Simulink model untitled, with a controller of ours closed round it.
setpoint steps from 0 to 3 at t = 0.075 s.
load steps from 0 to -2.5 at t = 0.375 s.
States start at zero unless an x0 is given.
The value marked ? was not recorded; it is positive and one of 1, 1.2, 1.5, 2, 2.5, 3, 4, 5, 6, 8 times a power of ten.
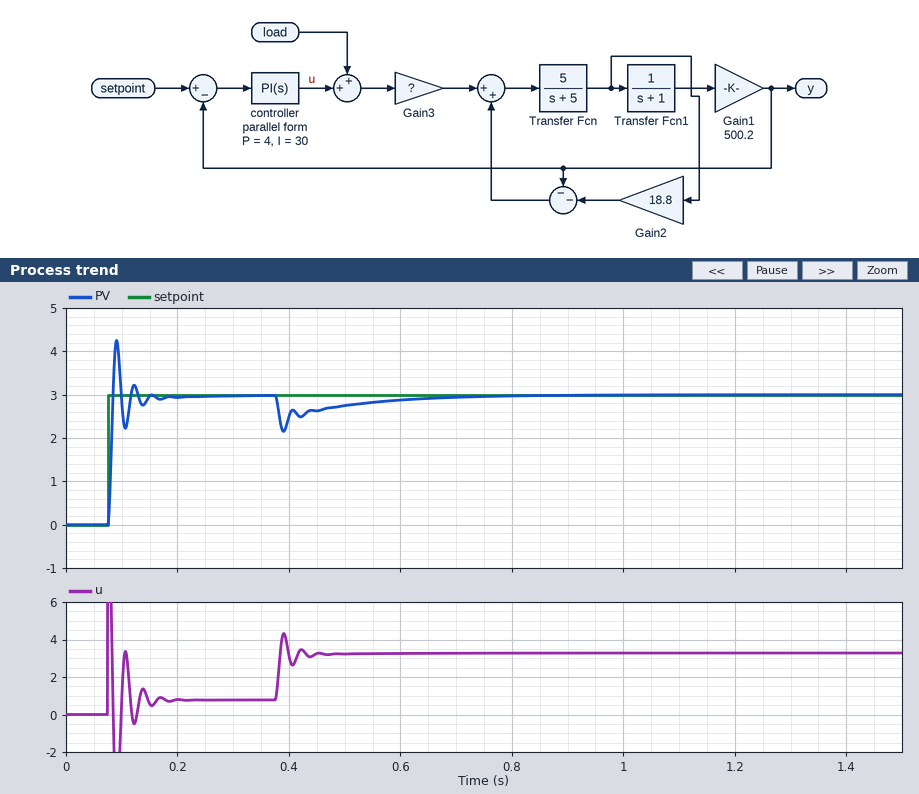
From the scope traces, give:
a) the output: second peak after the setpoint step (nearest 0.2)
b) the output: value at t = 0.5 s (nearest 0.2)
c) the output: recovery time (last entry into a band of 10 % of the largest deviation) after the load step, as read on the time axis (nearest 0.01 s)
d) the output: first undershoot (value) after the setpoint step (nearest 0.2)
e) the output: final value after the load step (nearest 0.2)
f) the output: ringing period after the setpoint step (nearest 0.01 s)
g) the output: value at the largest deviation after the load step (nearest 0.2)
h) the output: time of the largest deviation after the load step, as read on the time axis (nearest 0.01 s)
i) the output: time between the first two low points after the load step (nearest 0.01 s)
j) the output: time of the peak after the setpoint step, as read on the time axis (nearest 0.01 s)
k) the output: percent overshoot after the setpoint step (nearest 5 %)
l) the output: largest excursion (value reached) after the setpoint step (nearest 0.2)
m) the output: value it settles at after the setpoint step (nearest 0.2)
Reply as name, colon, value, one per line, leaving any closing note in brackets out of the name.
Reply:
the output: second peak after the setpoint step: 3.2
the output: value at t = 0.5 s: 2.8
the output: recovery time (last entry into a band of 10 % of the largest deviation) after the load step, as read on the time axis: 0.66 s
the output: first undershoot (value) after the setpoint step: 2.2
the output: final value after the load step: 3.0
the output: ringing period after the setpoint step: 0.03 s
the output: value at the largest deviation after the load step: 2.2
the output: time of the largest deviation after the load step, as read on the time axis: 0.39 s
the output: time between the first two low points after the load step: 0.03 s
the output: time of the peak after the setpoint step, as read on the time axis: 0.09 s
the output: percent overshoot after the setpoint step: 40 %
the output: largest excursion (value reached) after the setpoint step: 4.2
the output: value it settles at after the setpoint step: 3.0
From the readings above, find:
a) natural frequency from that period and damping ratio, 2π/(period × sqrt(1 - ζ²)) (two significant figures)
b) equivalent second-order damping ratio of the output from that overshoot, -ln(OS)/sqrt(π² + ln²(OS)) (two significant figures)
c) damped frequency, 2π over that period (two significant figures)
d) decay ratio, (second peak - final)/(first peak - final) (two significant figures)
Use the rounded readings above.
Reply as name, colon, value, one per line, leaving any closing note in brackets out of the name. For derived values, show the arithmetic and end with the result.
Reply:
natural frequency from that period and damping ratio, 2π/(period × sqrt(1 - ζ²)): 2π / (0.03 × sqrt(1 - 0.28²)) = 220 rad/s
equivalent second-order damping ratio of the output from that overshoot, -ln(OS)/sqrt(π² + ln²(OS)): ln(0.4) = -0.916; 0.916 / sqrt(9.870 + 0.840) = 0.28
damped frequency, 2π over that period: 2π / 0.03 = 210 rad/s
decay ratio, (second peak - final)/(first peak - final): (3.2 - 3) / (4.2 - 3) = 0.17
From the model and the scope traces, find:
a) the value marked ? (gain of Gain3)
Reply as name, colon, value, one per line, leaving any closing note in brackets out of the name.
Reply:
the value marked ?: 4
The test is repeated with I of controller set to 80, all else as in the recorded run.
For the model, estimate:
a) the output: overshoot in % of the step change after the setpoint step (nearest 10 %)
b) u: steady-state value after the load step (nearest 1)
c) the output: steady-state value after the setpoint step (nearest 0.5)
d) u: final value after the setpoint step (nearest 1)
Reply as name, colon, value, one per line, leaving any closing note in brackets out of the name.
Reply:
the output: overshoot in % of the step change after the setpoint step: 50 %
u: steady-state value after the load step: 3
the output: steady-state value after the setpoint step: 3.0
u: final value after the setpoint step: 1
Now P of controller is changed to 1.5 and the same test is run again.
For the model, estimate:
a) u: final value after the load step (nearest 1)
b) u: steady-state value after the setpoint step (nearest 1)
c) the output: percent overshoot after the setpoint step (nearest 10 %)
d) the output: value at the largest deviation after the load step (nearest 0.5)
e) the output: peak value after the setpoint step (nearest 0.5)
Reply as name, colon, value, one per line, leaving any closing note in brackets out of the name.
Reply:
u: final value after the load step: 3
u: steady-state value after the setpoint step: 1
the output: percent overshoot after the setpoint step: 30 %
the output: value at the largest deviation after the load step: 1.5
the output: peak value after the setpoint step: 4.0
